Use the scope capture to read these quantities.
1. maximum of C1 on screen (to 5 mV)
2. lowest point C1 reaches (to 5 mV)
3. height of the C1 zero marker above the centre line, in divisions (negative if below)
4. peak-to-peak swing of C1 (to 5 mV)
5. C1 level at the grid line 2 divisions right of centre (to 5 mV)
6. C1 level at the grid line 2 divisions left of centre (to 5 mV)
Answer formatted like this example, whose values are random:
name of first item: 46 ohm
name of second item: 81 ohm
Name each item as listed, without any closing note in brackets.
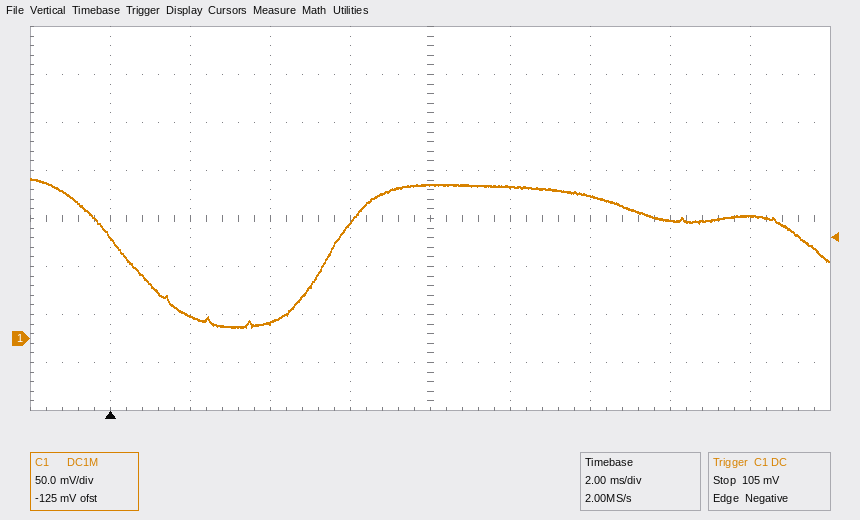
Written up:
maximum of C1 on screen: 165 mV
lowest point C1 reaches: 10 mV
height of the C1 zero marker above the centre line, in divisions: -2.5 div
peak-to-peak swing of C1: 155 mV
C1 level at the grid line 2 divisions right of centre: 150 mV
C1 level at the grid line 2 divisions left of centre: 15 mV
